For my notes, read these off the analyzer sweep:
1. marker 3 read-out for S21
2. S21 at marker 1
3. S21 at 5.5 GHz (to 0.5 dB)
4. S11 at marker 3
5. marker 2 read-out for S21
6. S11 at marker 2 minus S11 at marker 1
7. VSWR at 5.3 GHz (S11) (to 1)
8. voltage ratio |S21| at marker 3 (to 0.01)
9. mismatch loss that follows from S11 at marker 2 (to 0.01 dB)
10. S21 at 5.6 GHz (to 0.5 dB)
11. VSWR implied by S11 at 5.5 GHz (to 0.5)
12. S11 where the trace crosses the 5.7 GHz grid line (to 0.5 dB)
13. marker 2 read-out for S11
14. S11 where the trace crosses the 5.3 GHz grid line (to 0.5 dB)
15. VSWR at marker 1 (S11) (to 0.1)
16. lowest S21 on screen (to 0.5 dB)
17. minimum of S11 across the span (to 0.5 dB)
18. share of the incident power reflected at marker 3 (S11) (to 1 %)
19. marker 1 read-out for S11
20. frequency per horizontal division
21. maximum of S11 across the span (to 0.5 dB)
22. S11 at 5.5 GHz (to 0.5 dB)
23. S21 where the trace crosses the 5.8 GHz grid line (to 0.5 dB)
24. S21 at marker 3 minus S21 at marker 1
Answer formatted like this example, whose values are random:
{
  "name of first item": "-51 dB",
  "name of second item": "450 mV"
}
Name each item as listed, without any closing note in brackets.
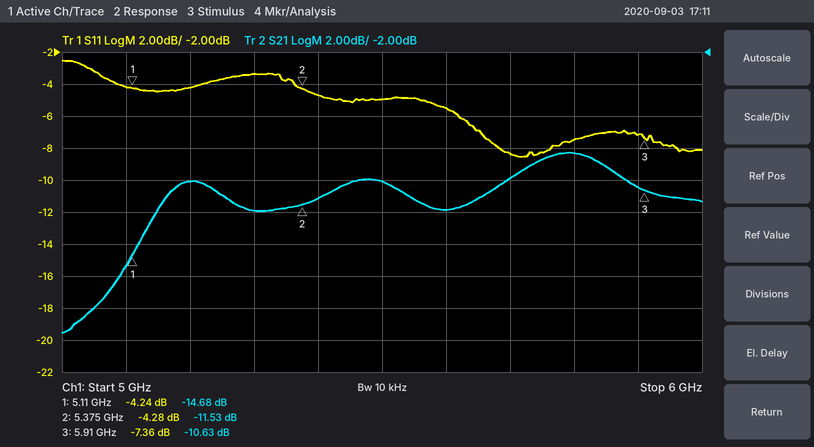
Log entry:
{
  "marker 3 read-out for S21": "-10.63 dB",
  "S21 at marker 1": "-14.68 dB",
  "S21 at 5.5 GHz": "-10.0 dB",
  "S11 at marker 3": "-7.36 dB",
  "marker 2 read-out for S21": "-11.53 dB",
  "S11 at marker 2 minus S11 at marker 1": "-0.04 dB",
  "VSWR at 5.3 GHz (S11)": "5",
  "voltage ratio |S21| at marker 3": "0.29",
  "mismatch loss that follows from S11 at marker 2": "2.03 dB",
  "S21 at 5.6 GHz": "-12.0 dB",
  "VSWR implied by S11 at 5.5 GHz": "3.5",
  "S11 where the trace crosses the 5.7 GHz grid line": "-8.5 dB",
  "marker 2 read-out for S11": "-4.28 dB",
  "S11 where the trace crosses the 5.3 GHz grid line": "-3.5 dB",
  "VSWR at marker 1 (S11)": "4.2",
  "lowest S21 on screen": "-19.5 dB",
  "minimum of S11 across the span": "-8.5 dB",
  "share of the incident power reflected at marker 3 (S11)": "18 %",
  "marker 1 read-out for S11": "-4.24 dB",
  "frequency per horizontal division": "100 MHz",
  "maximum of S11 across the span": "-2.5 dB",
  "S11 at 5.5 GHz": "-5.0 dB",
  "S21 where the trace crosses the 5.8 GHz grid line": "-8.5 dB",
  "S21 at marker 3 minus S21 at marker 1": "4.05 dB"
}
